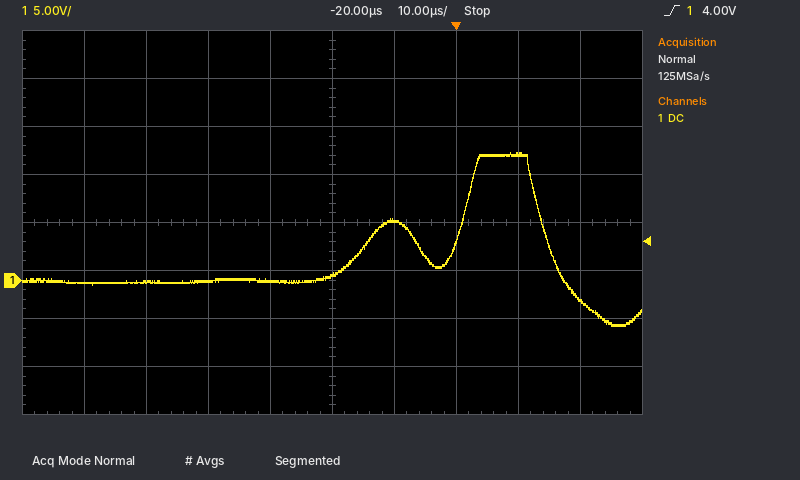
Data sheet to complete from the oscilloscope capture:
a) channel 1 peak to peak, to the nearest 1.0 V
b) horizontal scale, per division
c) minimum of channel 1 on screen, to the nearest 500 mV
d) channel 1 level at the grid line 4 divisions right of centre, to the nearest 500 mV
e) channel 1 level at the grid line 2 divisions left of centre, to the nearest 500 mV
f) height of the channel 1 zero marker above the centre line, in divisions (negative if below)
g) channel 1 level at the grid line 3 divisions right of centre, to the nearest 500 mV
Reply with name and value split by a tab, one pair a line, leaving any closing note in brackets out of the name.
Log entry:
channel 1 peak to peak, to the nearest 1.0 V	18.0 V
horizontal scale, per division	10 µs
minimum of channel 1 on screen, to the nearest 500 mV	-5.0 V
channel 1 level at the grid line 4 divisions right of centre, to the nearest 500 mV	-2.0 V
channel 1 level at the grid line 2 divisions left of centre, to the nearest 500 mV	0.0 V
height of the channel 1 zero marker above the centre line, in divisions	-1.2 div
channel 1 level at the grid line 3 divisions right of centre, to the nearest 500 mV	13.0 V
